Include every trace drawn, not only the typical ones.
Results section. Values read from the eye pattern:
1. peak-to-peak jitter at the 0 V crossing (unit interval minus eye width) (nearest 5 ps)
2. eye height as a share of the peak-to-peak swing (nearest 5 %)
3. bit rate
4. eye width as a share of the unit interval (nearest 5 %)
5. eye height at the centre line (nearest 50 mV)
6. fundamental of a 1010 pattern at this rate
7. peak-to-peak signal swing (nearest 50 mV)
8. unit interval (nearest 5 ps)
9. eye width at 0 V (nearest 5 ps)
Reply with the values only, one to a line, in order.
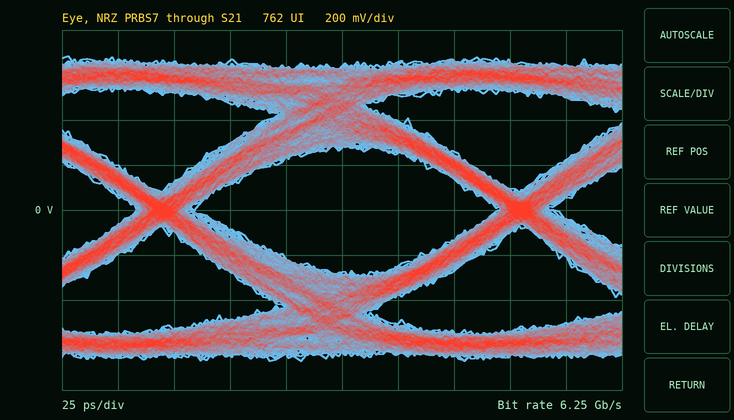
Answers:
25 ps
40 %
6.25 Gb/s
85 %
550 mV
3.125 GHz
1.35 V
160 ps
135 ps
